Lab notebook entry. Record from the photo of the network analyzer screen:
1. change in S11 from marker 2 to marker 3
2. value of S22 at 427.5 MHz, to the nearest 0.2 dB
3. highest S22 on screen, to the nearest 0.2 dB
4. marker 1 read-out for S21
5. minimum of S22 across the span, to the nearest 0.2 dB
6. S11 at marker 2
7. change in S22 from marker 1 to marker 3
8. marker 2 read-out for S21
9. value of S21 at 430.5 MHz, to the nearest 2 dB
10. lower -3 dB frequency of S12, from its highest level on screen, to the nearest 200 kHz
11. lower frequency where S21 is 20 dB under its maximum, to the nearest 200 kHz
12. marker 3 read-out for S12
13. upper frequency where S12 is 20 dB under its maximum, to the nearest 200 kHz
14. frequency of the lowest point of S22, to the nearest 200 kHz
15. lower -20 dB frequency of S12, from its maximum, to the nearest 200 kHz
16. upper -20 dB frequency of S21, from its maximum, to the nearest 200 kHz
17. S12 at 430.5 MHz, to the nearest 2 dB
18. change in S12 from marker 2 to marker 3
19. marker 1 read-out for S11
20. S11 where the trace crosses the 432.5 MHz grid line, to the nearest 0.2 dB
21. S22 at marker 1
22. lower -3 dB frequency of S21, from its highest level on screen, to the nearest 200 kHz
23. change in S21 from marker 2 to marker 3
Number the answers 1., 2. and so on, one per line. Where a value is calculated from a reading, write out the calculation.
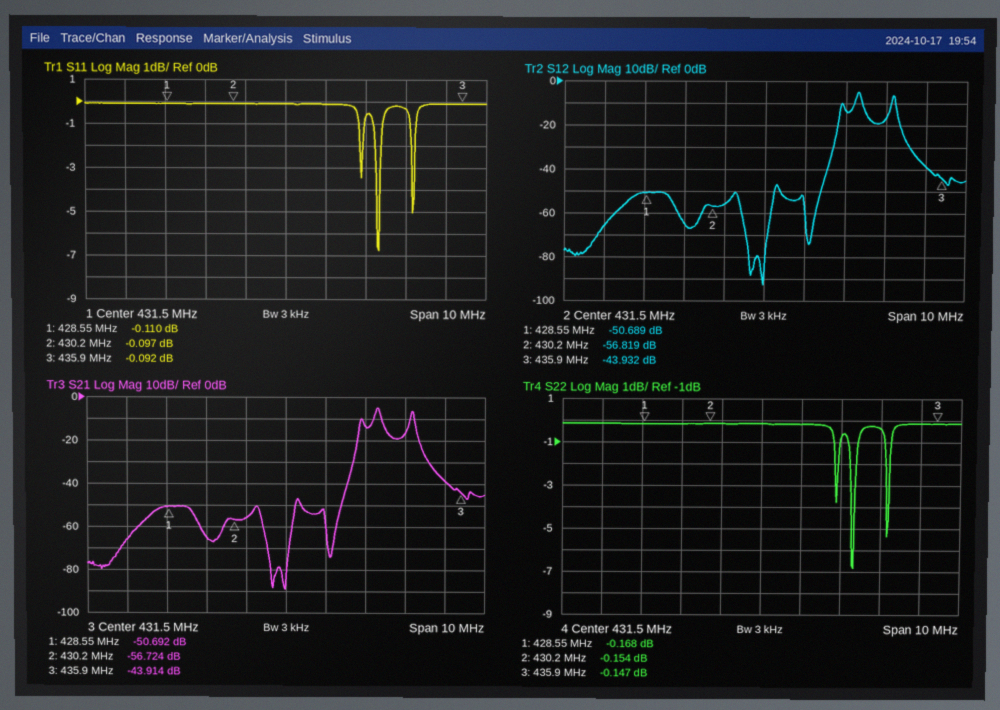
1. -0.092 − (-0.097) = 0.005 dB
2. -0.2 dB
3. -0.2 dB
4. -50.692 dB
5. -6.8 dB
6. -0.097 dB
7. -0.147 − (-0.168) = 0.021 dB
8. -56.724 dB
9. -56 dB
10. 433.8 MHz
11. 433.2 MHz
12. -43.932 dB
13. 435.0 MHz
14. 433.8 MHz
15. 433.2 MHz
16. 435.0 MHz
17. -56 dB
18. -43.932 − (-56.819) = 12.887 dB
19. -0.110 dB
20. -0.2 dB
21. -0.168 dB
22. 433.8 MHz
23. -43.914 − (-56.724) = 12.810 dB
